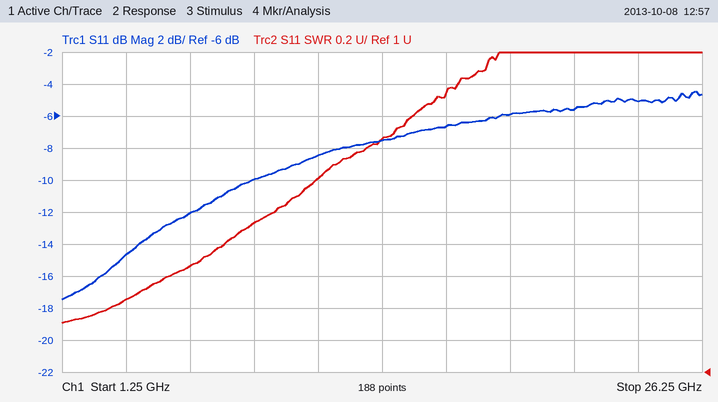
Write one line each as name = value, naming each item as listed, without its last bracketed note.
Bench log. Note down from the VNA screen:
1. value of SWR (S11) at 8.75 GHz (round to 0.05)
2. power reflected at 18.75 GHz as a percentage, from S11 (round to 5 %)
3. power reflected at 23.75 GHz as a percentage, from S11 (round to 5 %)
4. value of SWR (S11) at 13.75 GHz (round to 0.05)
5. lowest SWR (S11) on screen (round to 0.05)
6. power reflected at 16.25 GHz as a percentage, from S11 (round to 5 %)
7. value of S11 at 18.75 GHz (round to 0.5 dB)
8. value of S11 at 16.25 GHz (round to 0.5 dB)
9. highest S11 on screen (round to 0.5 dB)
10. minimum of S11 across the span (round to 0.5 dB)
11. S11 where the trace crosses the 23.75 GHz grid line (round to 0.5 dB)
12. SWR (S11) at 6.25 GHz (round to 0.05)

value of SWR (S11) at 8.75 GHz = 1.95
power reflected at 18.75 GHz as a percentage, from S11 = 25 %
power reflected at 23.75 GHz as a percentage, from S11 = 30 %
value of SWR (S11) at 13.75 GHz = 2.45
lowest SWR (S11) on screen = 1.30
power reflected at 16.25 GHz as a percentage, from S11 = 20 %
value of S11 at 18.75 GHz = -6.0 dB
value of S11 at 16.25 GHz = -6.5 dB
highest S11 on screen = -4.5 dB
minimum of S11 across the span = -17.5 dB
S11 where the trace crosses the 23.75 GHz grid line = -5.0 dB
SWR (S11) at 6.25 GHz = 1.65
